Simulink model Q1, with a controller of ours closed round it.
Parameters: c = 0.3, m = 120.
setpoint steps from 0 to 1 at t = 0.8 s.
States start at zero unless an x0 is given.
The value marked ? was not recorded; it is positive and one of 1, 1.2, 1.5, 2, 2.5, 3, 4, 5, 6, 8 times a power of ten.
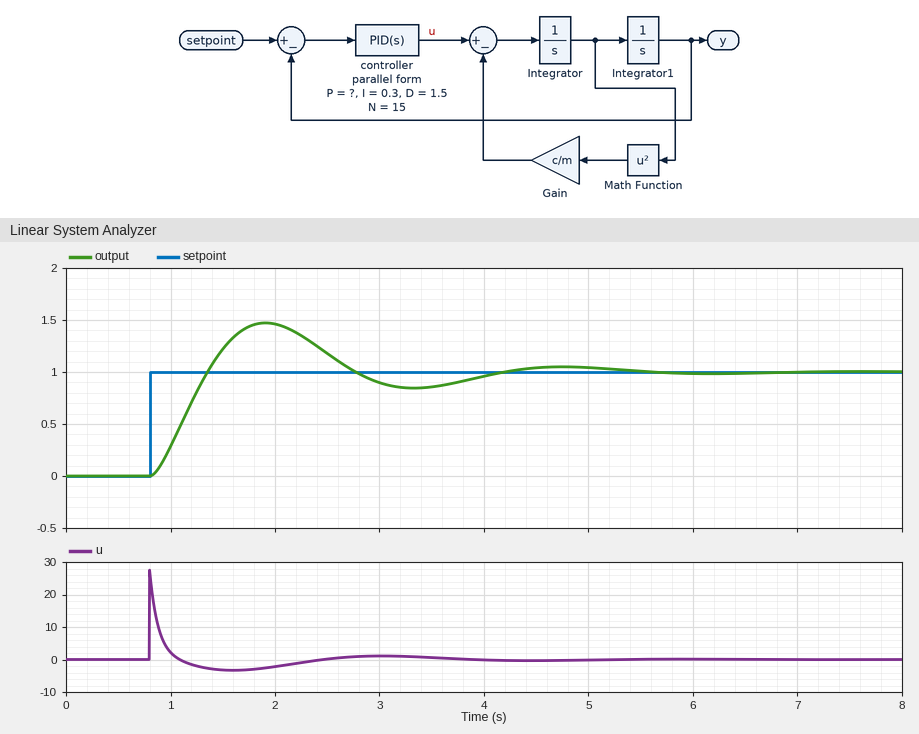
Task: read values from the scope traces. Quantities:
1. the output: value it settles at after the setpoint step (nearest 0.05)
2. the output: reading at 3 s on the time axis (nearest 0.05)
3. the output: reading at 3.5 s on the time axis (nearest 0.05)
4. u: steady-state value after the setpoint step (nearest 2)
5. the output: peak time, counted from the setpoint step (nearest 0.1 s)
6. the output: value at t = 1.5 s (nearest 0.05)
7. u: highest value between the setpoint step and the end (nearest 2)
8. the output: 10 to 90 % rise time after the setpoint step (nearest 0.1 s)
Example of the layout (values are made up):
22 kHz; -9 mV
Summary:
1.00; 0.90; 0.85; 0; 1.1 s; 1.20; 28; 0.4 s
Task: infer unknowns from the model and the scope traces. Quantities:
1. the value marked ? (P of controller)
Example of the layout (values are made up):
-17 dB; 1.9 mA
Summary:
5
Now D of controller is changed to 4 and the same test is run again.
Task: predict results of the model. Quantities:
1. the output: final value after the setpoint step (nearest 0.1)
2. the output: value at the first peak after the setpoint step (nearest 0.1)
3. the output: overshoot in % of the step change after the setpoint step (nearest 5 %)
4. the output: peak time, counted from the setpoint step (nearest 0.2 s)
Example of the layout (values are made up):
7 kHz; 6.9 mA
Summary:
1.0; 1.2; 20 %; 0.8 s
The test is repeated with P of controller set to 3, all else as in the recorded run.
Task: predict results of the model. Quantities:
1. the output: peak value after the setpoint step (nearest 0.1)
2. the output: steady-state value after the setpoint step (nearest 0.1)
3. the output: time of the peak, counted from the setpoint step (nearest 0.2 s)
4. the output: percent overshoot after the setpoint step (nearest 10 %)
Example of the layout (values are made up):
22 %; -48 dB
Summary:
1.4; 1.0; 1.4 s; 40 %
